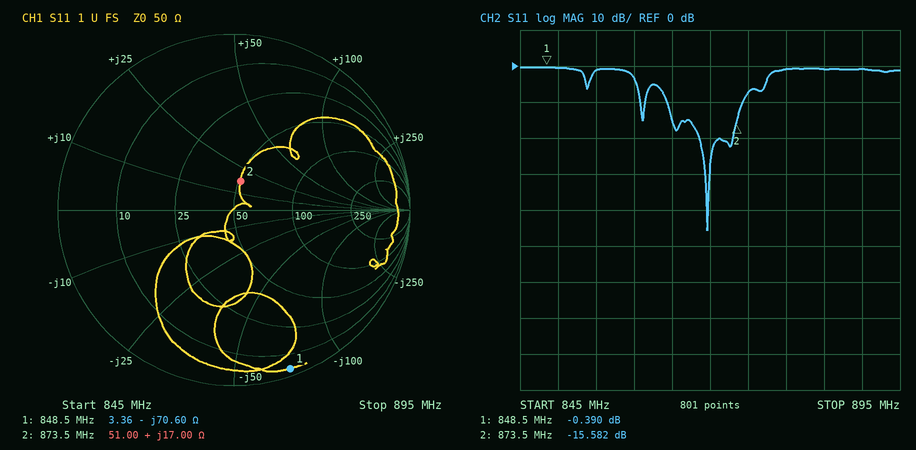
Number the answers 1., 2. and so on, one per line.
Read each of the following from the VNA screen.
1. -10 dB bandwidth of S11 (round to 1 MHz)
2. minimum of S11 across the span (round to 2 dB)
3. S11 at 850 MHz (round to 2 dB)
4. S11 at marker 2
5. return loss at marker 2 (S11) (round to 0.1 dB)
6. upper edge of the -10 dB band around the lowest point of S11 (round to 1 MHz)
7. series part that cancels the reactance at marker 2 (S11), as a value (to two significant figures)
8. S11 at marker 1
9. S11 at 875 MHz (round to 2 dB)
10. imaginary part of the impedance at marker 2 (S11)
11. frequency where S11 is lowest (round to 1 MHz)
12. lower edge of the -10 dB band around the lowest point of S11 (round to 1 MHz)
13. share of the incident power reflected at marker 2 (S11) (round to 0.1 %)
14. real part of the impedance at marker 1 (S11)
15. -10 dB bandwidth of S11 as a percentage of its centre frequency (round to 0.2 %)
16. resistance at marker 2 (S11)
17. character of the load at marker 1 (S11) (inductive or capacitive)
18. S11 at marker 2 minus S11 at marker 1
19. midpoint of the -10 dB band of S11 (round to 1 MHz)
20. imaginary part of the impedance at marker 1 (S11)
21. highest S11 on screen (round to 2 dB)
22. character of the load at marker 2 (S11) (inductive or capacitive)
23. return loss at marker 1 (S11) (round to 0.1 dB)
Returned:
1. 10 MHz
2. -46 dB
3. 0 dB
4. -15.582 dB
5. 15.6 dB
6. 874 MHz
7. 11 pF
8. -0.390 dB
9. -8 dB
10. +17.00 Ω
11. 870 MHz
12. 864 MHz
13. 2.8 %
14. 3.36 Ω
15. 1.2 %
16. 51.00 Ω
17. capacitive
18. -15.192 dB
19. 869 MHz
20. -70.60 Ω
21. 0 dB
22. inductive
23. 0.4 dB
